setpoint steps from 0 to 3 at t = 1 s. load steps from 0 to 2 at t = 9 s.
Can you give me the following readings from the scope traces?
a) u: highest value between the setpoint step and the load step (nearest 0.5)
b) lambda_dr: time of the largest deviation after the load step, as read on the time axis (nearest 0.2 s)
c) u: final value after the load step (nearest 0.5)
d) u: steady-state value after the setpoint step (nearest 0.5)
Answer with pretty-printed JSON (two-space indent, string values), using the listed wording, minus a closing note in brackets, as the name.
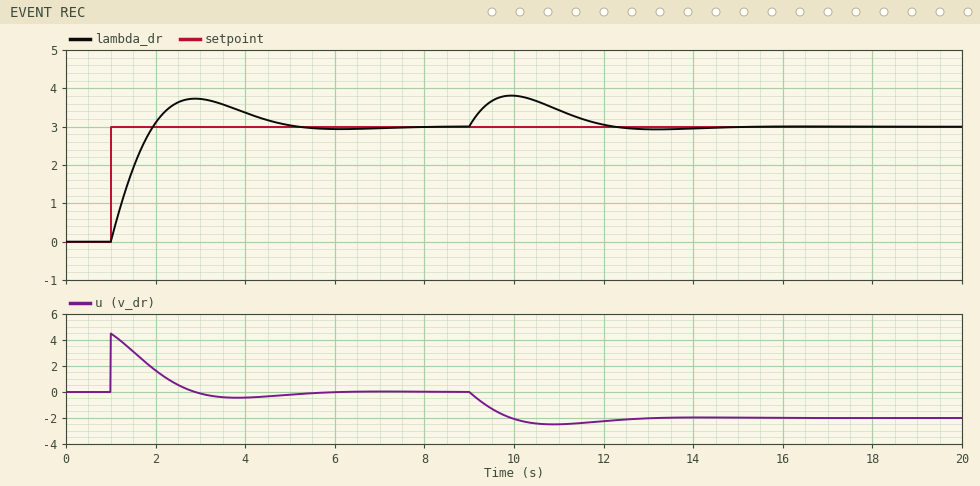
{
  "u: highest value between the setpoint step and the load step": "4.5",
  "lambda_dr: time of the largest deviation after the load step, as read on the time axis": "10.0 s",
  "u: final value after the load step": "-2.0",
  "u: steady-state value after the setpoint step": "0.0"
}
